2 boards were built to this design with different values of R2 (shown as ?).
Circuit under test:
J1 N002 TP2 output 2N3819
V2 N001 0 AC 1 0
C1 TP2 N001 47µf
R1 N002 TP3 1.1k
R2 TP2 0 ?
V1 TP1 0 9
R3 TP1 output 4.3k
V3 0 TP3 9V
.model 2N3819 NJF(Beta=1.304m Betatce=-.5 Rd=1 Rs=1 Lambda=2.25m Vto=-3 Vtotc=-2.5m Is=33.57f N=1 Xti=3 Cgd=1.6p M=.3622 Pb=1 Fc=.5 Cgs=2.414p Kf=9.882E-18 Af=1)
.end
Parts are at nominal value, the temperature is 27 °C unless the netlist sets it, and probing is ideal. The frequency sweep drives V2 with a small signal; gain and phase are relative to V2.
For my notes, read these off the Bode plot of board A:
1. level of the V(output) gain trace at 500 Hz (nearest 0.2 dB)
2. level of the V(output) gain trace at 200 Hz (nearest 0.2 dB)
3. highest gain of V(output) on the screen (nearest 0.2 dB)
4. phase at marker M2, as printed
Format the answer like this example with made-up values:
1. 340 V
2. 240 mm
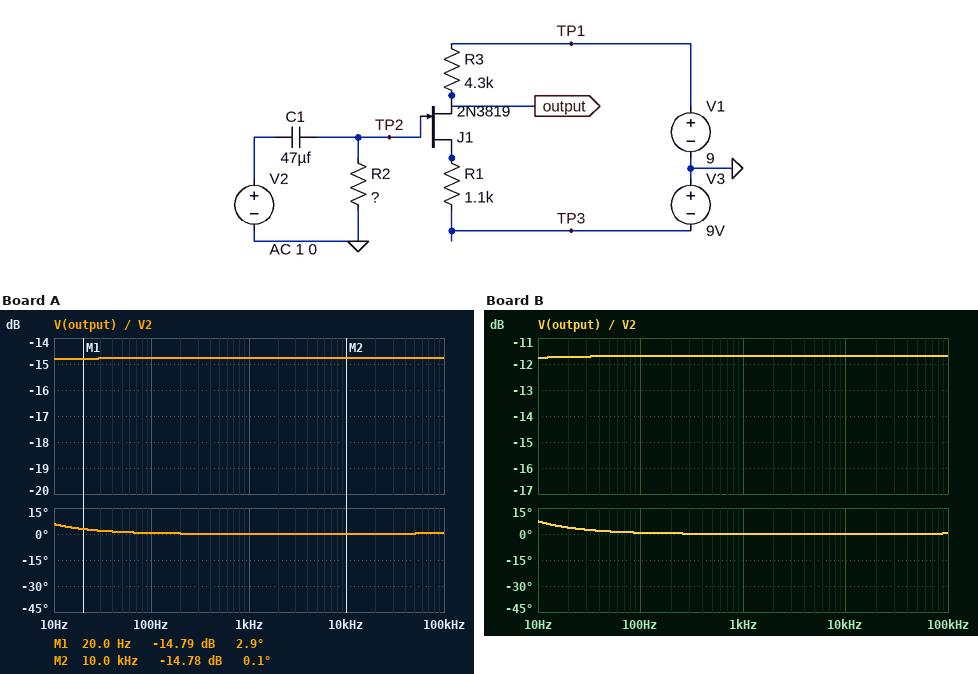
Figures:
1. -14.8 dB
2. -14.8 dB
3. -14.8 dB
4. 0.1 deg
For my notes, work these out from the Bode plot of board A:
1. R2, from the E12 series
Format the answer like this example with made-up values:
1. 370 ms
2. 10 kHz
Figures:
1. 470 kΩ
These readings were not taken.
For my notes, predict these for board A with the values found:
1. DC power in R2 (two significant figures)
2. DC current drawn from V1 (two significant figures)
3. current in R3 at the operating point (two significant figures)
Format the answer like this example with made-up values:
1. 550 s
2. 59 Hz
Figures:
1. 51 µW
2. 3.3 mA
3. 3.3 mA
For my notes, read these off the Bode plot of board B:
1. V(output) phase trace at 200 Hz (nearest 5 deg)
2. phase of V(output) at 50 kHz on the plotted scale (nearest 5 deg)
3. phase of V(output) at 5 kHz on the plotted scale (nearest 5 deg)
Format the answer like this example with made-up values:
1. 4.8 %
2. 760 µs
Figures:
1. 0 deg
2. 0 deg
3. 0 deg
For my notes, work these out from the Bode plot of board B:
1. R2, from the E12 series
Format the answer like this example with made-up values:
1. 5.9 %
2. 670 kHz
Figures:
1. 330 kΩ
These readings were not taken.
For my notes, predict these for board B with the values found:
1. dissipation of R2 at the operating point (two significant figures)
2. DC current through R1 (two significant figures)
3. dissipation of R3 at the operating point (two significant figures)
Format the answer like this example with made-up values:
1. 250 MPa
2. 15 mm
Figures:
1. 72 µW
2. 3.3 mA
3. 46 mW
